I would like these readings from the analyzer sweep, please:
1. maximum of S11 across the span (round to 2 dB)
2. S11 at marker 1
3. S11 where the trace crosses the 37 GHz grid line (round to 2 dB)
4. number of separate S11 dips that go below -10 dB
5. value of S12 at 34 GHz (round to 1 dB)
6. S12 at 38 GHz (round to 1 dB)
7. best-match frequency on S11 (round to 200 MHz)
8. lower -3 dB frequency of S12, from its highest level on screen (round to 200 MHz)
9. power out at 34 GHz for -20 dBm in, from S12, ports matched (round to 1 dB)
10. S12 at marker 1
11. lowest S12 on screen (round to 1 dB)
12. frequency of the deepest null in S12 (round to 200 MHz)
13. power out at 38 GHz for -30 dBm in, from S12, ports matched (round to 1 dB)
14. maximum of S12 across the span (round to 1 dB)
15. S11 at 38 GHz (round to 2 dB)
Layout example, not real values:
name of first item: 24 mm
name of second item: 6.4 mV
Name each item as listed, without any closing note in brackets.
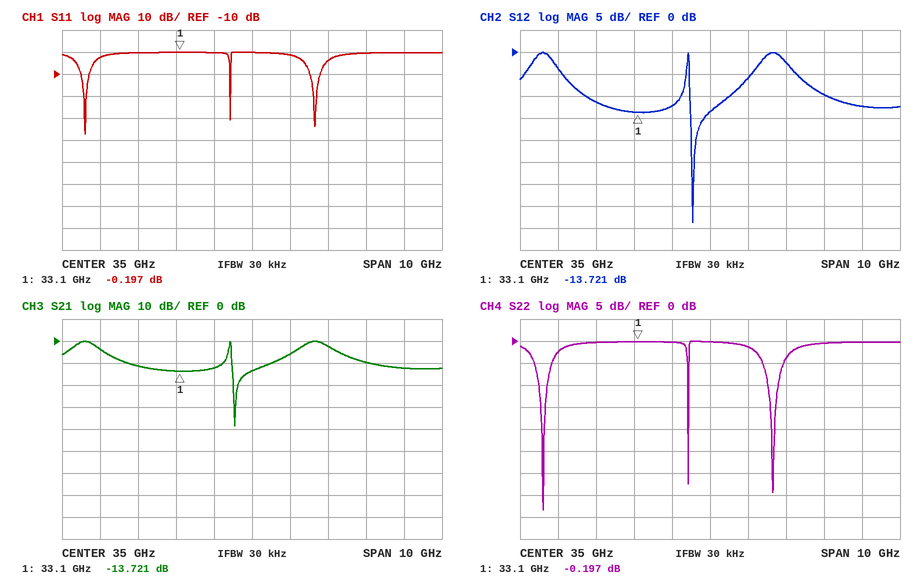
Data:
maximum of S11 across the span: 0 dB
S11 at marker 1: -0.197 dB
S11 where the trace crosses the 37 GHz grid line: -4 dB
number of separate S11 dips that go below -10 dB: 3
value of S12 at 34 GHz: -12 dB
S12 at 38 GHz: -10 dB
best-match frequency on S11: 30.6 GHz
lower -3 dB frequency of S12, from its highest level on screen: 30.2 GHz
power out at 34 GHz for -20 dBm in, from S12, ports matched: -32 dBm
S12 at marker 1: -13.721 dB
lowest S12 on screen: -39 dB
frequency of the deepest null in S12: 34.6 GHz
power out at 38 GHz for -30 dBm in, from S12, ports matched: -40 dBm
maximum of S12 across the span: 0 dB
S11 at 38 GHz: 0 dB
